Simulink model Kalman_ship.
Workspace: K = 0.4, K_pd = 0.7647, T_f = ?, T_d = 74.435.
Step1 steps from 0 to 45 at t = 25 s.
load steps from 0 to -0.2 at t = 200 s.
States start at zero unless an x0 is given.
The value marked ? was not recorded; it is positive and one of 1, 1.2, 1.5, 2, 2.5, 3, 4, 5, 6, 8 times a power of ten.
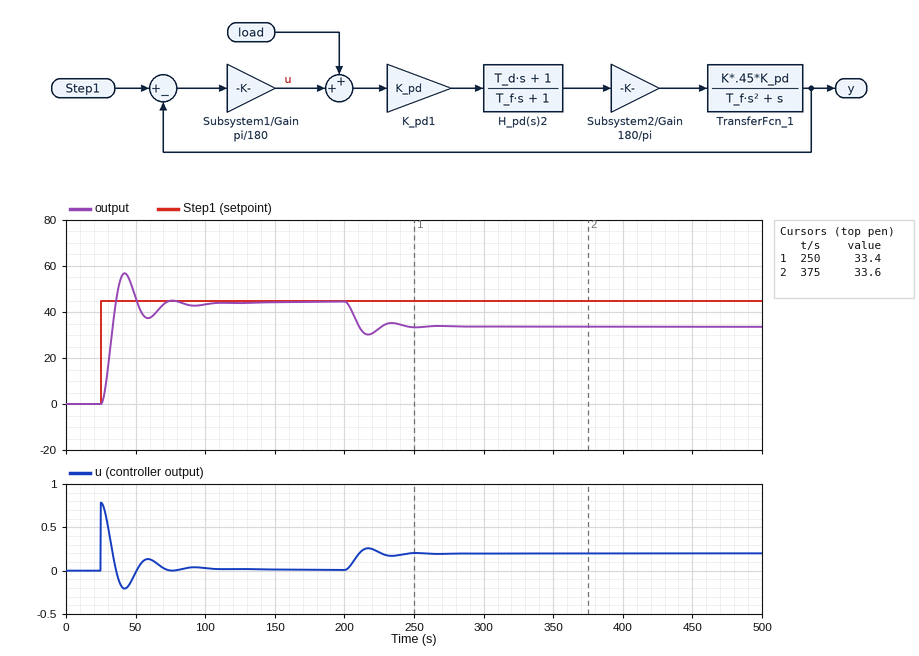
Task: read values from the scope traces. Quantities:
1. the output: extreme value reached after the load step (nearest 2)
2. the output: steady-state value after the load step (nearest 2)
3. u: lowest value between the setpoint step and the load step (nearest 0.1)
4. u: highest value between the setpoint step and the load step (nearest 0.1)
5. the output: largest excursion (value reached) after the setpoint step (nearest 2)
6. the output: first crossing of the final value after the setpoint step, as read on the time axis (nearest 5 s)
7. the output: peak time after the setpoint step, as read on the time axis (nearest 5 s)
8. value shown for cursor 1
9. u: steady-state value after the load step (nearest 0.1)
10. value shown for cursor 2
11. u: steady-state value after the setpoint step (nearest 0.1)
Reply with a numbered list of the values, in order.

1. 30
2. 34
3. -0.2
4. 0.8
5. 56
6. 35 s
7. 40 s
8. 33.4
9. 0.2
10. 33.6
11. 0.0
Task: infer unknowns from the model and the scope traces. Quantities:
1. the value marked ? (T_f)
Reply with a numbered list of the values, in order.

1. 15
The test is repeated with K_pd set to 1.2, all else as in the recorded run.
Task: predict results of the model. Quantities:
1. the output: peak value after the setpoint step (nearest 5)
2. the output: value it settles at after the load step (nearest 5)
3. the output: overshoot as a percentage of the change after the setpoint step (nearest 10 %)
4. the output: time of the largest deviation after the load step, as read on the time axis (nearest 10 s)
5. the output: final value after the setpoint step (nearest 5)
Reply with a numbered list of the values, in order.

1. 65
2. 35
3. 50 %
4. 210 s
5. 45
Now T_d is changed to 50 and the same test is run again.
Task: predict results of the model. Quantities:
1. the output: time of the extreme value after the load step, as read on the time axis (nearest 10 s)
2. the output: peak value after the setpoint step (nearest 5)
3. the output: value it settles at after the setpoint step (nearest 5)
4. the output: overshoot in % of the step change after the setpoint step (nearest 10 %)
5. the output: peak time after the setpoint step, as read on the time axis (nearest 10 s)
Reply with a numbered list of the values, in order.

1. 220 s
2. 55
3. 45
4. 20 %
5. 50 s
